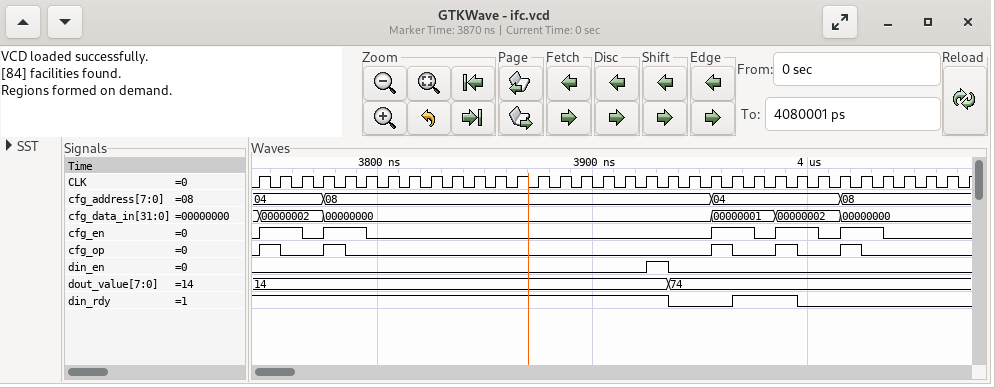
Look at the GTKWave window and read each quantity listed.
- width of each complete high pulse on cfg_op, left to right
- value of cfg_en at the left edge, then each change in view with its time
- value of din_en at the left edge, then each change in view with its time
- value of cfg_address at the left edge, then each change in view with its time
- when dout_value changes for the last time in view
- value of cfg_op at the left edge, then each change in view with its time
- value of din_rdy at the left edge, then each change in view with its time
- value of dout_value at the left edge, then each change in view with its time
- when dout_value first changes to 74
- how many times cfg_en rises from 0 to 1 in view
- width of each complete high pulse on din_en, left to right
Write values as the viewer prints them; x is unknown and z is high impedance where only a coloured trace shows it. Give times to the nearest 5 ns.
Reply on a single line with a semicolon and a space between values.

10 ns, 10 ns, 10 ns, 10 ns, 10 ns; 0, 1 at 3745 ns, 0 at 3765 ns, 1 at 3775 ns, 0 at 3795 ns, 1 at 3955 ns, 0 at 3975 ns, 1 at 3985 ns, 0 at 4005 ns, 1 at 4015 ns, 0 at 4035 ns; 0, 1 at 3925 ns, 0 at 3935 ns; 04, 08 at 3775 ns, 04 at 3955 ns, 08 at 4015 ns; 3935 ns; 0, 1 at 3745 ns, 0 at 3755 ns, 1 at 3775 ns, 0 at 3785 ns, 1 at 3955 ns, 0 at 3965 ns, 1 at 3985 ns, 0 at 3995 ns, 1 at 4015 ns, 0 at 4025 ns; 1, 0 at 3935 ns, 1 at 3965 ns, 0 at 3995 ns; 14, 74 at 3935 ns; 3935 ns; 5; 10 ns
